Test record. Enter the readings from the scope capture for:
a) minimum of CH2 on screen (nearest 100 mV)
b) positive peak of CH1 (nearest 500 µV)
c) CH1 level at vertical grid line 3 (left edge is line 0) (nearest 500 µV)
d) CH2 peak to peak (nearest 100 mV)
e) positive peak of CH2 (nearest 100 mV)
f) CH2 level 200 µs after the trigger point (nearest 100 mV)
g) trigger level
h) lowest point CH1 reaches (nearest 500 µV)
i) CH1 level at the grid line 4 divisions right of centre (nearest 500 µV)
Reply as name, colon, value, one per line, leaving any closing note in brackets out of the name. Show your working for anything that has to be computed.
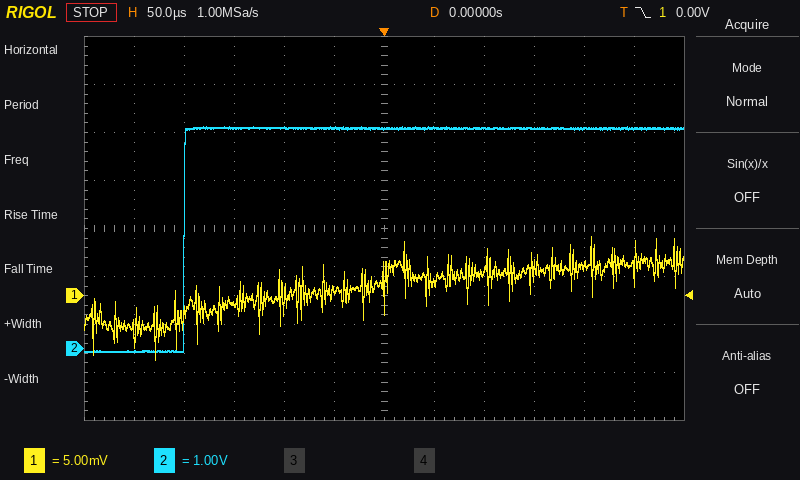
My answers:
minimum of CH2 on screen: -100 mV
positive peak of CH1: 6.0 mV
CH1 level at vertical grid line 3 (left edge is line 0): -500 µV
CH2 peak to peak: 4.6 V − (-100 mV) = 4.7 V
positive peak of CH2: 4.6 V
CH2 level 200 µs after the trigger point: 4.6 V
trigger level: 0.00 V
lowest point CH1 reaches: -6.5 mV
CH1 level at the grid line 4 divisions right of centre: 3.0 mV
